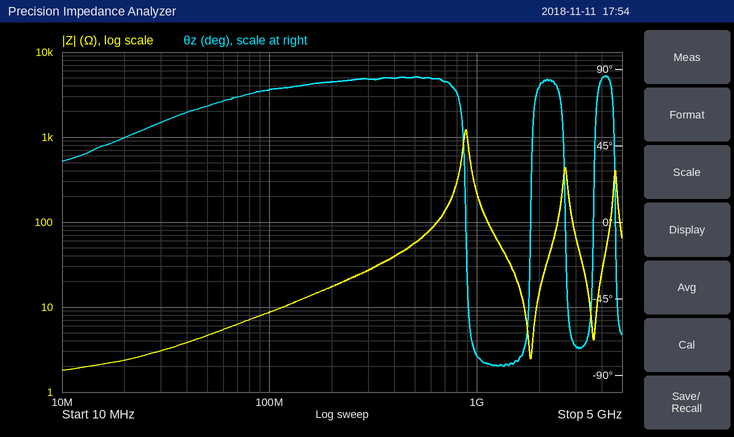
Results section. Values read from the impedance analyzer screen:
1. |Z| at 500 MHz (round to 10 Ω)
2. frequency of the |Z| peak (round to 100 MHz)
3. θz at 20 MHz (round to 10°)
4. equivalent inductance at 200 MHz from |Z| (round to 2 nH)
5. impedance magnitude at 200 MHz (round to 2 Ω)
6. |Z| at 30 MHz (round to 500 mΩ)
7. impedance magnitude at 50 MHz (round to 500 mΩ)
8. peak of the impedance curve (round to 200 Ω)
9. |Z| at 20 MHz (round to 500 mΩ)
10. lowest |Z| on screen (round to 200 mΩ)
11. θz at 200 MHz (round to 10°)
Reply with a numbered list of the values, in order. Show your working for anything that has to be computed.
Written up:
1. 60 Ω
2. 900 MHz
3. 50°
4. L = 18 Ω/(2π × 200 MHz) ≈ 14 nH
5. 18 Ω
6. 3.0 Ω
7. 4.5 Ω
8. 1.2 kΩ
9. 2.5 Ω
10. 1.8 Ω
11. 80°
